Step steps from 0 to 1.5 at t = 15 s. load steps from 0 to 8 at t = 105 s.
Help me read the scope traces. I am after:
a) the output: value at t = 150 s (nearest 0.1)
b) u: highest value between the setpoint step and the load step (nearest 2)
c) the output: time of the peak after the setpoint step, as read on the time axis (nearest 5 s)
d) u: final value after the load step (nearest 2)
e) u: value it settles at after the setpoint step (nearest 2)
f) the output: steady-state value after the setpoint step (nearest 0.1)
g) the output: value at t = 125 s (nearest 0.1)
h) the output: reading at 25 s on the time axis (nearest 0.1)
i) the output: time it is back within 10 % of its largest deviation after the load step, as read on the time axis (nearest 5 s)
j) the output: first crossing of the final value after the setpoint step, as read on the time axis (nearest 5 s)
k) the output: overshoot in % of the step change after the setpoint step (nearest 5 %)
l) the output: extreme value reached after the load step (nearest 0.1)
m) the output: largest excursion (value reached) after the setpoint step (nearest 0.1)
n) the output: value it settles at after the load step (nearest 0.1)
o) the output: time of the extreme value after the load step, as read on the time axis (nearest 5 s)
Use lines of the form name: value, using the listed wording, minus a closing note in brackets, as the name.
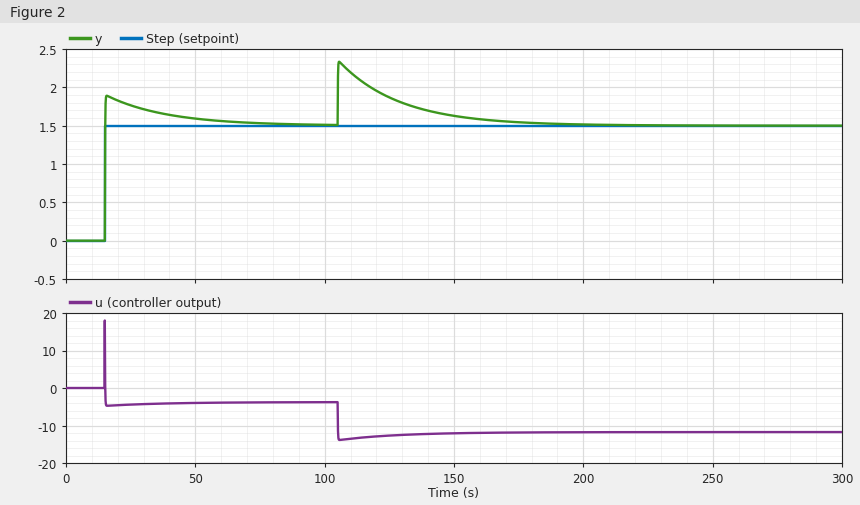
the output: value at t = 150 s: 1.6
u: highest value between the setpoint step and the load step: 18
the output: time of the peak after the setpoint step, as read on the time axis: 15 s
u: final value after the load step: -12
u: value it settles at after the setpoint step: -4
the output: steady-state value after the setpoint step: 1.5
the output: value at t = 125 s: 1.9
the output: reading at 25 s on the time axis: 1.8
the output: time it is back within 10 % of its largest deviation after the load step, as read on the time axis: 160 s
the output: first crossing of the final value after the setpoint step, as read on the time axis: 15 s
the output: overshoot in % of the step change after the setpoint step: 25 %
the output: extreme value reached after the load step: 2.3
the output: largest excursion (value reached) after the setpoint step: 1.9
the output: value it settles at after the load step: 1.5
the output: time of the extreme value after the load step, as read on the time axis: 105 s
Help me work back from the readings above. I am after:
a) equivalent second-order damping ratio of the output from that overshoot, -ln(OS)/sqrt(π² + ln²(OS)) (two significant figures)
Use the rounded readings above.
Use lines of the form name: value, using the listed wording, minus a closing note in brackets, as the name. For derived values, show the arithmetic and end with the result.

equivalent second-order damping ratio of the output from that overshoot, -ln(OS)/sqrt(π² + ln²(OS)): ln(0.25) = -1.386; 1.386 / sqrt(9.870 + 1.922) = 0.40
